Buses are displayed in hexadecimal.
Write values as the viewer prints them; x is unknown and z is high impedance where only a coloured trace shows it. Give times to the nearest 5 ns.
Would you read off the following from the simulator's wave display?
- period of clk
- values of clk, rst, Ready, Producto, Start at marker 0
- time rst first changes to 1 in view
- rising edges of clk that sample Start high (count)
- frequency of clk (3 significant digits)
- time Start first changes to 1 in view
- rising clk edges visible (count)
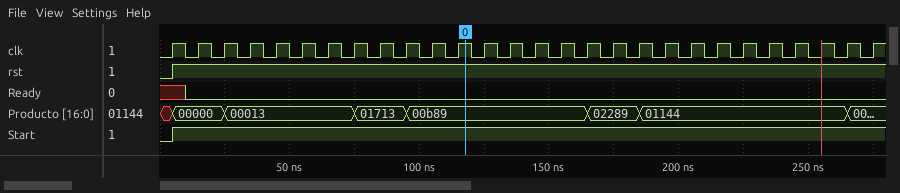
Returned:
10 ns
clk=1, rst=1, Ready=0, Producto=00b89, Start=1
5 ns
27
100 MHz
5 ns
28
